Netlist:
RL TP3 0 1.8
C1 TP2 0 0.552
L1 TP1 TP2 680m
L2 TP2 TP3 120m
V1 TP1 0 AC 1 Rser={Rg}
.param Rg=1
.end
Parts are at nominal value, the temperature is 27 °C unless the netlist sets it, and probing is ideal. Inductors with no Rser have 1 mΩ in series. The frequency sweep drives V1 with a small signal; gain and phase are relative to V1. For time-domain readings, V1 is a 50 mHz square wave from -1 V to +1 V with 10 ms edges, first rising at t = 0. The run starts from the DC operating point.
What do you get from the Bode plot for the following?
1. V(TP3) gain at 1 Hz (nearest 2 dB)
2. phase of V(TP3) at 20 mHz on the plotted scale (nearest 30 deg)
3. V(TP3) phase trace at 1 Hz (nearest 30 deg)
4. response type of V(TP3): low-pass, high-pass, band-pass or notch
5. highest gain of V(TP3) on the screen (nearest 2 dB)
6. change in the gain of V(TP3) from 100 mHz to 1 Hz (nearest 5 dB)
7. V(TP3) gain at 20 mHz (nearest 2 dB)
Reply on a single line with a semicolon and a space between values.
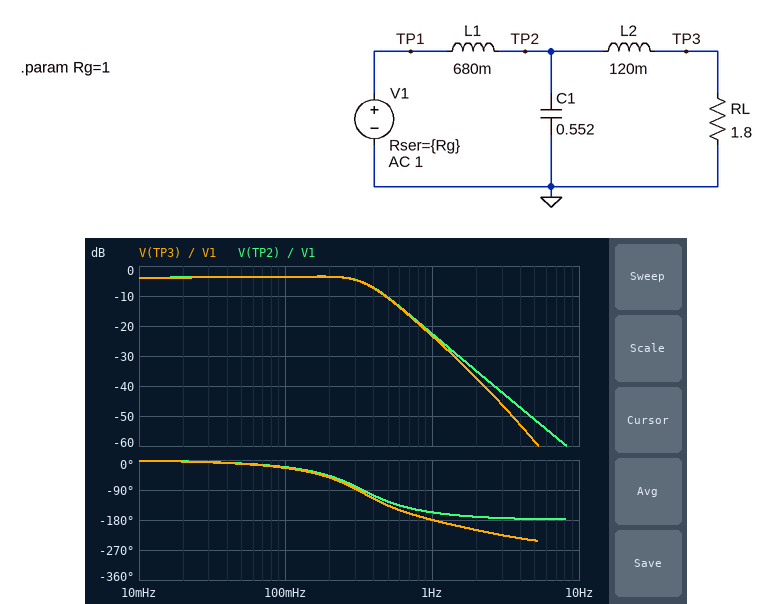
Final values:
-24 dB; 0 deg; -180 deg; low-pass; -4 dB; -20 dB; -4 dB
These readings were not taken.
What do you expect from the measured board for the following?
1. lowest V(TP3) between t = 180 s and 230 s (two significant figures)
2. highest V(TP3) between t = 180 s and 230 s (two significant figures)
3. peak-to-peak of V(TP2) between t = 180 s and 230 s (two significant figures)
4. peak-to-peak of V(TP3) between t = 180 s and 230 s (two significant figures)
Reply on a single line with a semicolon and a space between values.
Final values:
-760 mV; 760 mV; 1.5 V; 1.5 V
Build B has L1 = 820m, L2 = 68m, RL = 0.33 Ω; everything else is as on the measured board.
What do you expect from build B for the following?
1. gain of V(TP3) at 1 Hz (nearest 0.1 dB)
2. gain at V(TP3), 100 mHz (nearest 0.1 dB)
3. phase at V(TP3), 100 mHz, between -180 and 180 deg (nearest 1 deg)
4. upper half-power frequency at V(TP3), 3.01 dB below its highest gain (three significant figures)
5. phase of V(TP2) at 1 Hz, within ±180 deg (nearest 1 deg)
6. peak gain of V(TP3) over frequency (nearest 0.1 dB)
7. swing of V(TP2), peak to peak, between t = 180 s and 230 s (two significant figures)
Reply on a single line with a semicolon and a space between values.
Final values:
-25.4 dB; -12.7 dB; -28 deg; 283 mHz; -136 deg; -12.1 dB; 500 mV
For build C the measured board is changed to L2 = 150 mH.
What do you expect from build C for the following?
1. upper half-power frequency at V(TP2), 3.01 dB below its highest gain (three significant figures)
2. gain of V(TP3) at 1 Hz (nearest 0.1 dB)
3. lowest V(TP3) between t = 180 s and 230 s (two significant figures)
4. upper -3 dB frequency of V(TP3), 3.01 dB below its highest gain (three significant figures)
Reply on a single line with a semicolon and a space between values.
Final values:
378 mHz; -23.6 dB; -760 mV; 374 mHz
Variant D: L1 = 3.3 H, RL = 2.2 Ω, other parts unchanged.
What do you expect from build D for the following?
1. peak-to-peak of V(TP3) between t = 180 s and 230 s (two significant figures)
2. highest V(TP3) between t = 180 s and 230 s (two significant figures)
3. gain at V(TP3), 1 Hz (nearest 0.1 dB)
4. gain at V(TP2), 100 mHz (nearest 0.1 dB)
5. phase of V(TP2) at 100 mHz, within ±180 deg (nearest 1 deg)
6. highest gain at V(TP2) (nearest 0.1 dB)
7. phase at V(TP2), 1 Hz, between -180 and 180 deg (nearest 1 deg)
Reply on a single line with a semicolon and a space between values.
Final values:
1.6 V; 790 mV; -37.2 dB; -3.4 dB; -59 deg; -3.1 dB; -170 deg
